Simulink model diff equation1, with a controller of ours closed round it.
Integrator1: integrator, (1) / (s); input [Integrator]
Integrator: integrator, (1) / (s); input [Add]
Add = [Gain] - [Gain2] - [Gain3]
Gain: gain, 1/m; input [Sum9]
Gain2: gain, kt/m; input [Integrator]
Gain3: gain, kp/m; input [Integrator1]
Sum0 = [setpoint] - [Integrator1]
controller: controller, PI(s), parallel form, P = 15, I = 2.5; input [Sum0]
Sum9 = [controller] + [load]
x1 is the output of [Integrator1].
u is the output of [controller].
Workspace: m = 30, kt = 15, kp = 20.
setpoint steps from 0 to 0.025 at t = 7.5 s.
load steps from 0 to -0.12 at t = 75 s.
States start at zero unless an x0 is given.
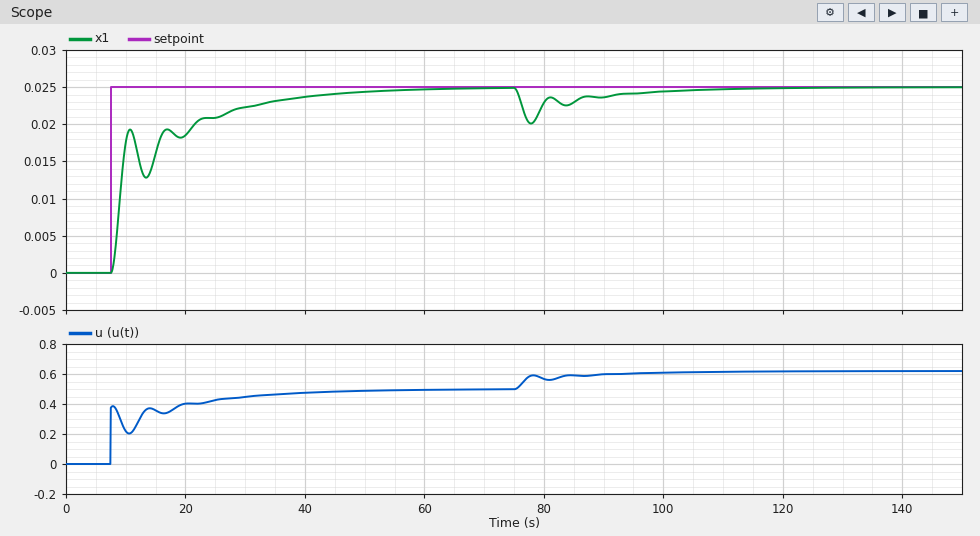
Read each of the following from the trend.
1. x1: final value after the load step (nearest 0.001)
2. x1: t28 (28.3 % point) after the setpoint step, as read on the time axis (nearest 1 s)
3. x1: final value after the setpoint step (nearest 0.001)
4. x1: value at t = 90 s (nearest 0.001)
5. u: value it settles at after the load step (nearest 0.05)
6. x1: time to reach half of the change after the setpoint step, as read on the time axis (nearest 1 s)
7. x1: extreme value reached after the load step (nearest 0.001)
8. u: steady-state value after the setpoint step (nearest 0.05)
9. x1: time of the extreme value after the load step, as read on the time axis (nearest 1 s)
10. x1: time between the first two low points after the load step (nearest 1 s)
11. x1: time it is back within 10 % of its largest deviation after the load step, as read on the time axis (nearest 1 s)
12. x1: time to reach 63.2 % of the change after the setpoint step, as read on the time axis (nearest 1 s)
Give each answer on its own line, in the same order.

0.025
9 s
0.025
0.024
0.60
9 s
0.020
0.50
78 s
6 s
103 s
10 s
